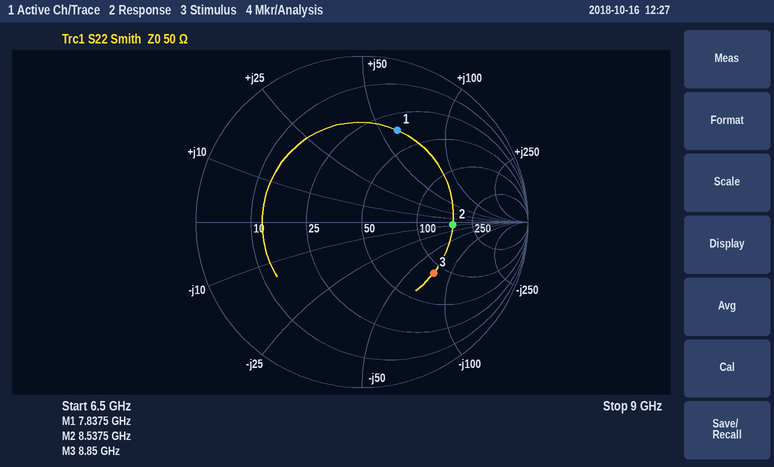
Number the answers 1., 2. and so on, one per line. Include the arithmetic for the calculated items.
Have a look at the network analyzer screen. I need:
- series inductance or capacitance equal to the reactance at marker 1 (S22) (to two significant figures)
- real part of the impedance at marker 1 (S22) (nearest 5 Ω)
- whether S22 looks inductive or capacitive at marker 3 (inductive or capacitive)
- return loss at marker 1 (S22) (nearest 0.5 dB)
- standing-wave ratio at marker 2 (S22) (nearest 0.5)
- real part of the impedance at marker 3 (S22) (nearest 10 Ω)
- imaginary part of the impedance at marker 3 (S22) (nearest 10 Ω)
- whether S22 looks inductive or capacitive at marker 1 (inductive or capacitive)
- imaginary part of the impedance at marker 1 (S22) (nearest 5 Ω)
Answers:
1. L = 60 Ω/(2π × 7.8375 GHz) ≈ 1.2 nH
2. 35 Ω
3. capacitive
4. 4.5 dB
5. 3.5
6. 90 Ω
7. -70 Ω
8. inductive
9. +60 Ω
